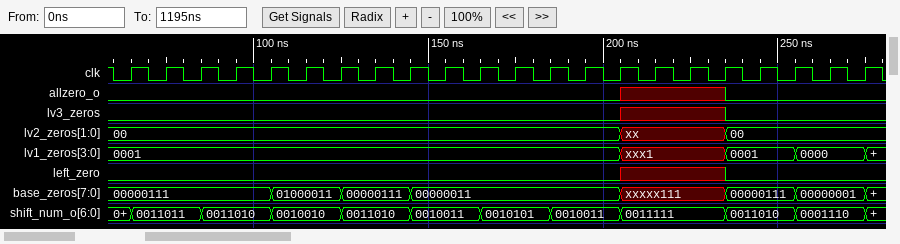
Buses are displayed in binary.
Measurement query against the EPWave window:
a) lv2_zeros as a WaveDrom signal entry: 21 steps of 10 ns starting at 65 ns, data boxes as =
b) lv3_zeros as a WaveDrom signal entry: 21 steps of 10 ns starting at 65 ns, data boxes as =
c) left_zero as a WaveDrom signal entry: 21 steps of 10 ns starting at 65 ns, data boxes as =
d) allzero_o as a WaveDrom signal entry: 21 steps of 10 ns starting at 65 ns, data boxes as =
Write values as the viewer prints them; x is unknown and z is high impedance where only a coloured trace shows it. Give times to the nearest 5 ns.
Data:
{name: 'lv2_zeros', wave: '=.............x..=...', data: '00 00'}
{name: 'lv3_zeros', wave: '0.............x..0...'}
{name: 'left_zero', wave: '0.............x..0...'}
{name: 'allzero_o', wave: '0.............x..0...'}
